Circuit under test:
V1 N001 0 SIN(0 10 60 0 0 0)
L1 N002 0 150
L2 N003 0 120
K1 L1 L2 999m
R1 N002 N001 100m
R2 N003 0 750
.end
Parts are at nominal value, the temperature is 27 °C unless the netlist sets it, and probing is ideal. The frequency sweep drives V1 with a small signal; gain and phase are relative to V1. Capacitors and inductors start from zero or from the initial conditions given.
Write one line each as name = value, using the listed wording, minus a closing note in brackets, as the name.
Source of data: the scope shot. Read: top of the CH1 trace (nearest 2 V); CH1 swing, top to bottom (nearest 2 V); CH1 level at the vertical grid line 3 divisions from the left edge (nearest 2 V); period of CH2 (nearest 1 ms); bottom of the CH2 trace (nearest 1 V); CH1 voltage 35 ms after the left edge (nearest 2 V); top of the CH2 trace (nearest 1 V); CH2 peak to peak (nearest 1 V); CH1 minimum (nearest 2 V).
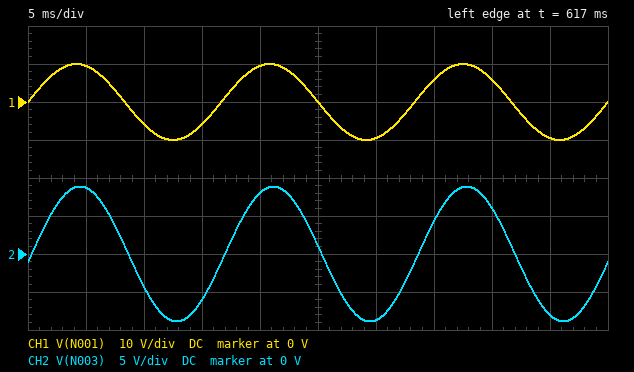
top of the CH1 trace = 10 V
CH1 swing, top to bottom = 20 V
CH1 level at the vertical grid line 3 divisions from the left edge = -6 V
period of CH2 = 17 ms
bottom of the CH2 trace = -9 V
CH1 voltage 35 ms after the left edge = 6 V
top of the CH2 trace = 9 V
CH2 peak to peak = 18 V
CH1 minimum = -10 V
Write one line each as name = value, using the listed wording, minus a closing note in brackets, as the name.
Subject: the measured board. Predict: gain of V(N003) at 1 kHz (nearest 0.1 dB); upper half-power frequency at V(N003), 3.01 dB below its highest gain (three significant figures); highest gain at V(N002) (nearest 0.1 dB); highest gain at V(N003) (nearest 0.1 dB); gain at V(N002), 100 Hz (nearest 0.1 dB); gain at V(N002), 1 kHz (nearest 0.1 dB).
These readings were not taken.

gain of V(N003) at 1 kHz = -8.0 dB
upper half-power frequency at V(N003), 3.01 dB below its highest gain = 498 Hz
highest gain at V(N002) = 0 dB
highest gain at V(N003) = -1.0 dB
gain at V(N002), 100 Hz = 0 dB
gain at V(N002), 1 kHz = 0 dB
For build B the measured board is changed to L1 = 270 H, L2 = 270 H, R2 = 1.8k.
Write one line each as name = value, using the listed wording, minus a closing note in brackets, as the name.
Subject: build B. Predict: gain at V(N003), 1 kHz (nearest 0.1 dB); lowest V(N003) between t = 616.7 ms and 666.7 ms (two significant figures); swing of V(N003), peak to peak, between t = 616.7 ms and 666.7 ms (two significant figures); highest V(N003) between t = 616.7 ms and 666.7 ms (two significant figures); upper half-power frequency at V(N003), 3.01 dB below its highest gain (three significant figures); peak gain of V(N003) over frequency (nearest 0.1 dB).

gain at V(N003), 1 kHz = -6.6 dB
lowest V(N003) between t = 616.7 ms and 666.7 ms = -9.9 V
swing of V(N003), peak to peak, between t = 616.7 ms and 666.7 ms = 20 V
highest V(N003) between t = 616.7 ms and 666.7 ms = 9.9 V
upper half-power frequency at V(N003), 3.01 dB below its highest gain = 531 Hz
peak gain of V(N003) over frequency = 0 dB
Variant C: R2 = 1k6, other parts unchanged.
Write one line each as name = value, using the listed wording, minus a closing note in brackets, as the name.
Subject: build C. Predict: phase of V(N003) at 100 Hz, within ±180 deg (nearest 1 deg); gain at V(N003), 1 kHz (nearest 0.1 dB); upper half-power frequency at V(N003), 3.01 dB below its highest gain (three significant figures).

phase of V(N003) at 100 Hz, within ±180 deg = -5 deg
gain at V(N003), 1 kHz = -3.7 dB
upper half-power frequency at V(N003), 3.01 dB below its highest gain = 1.06 kHz
